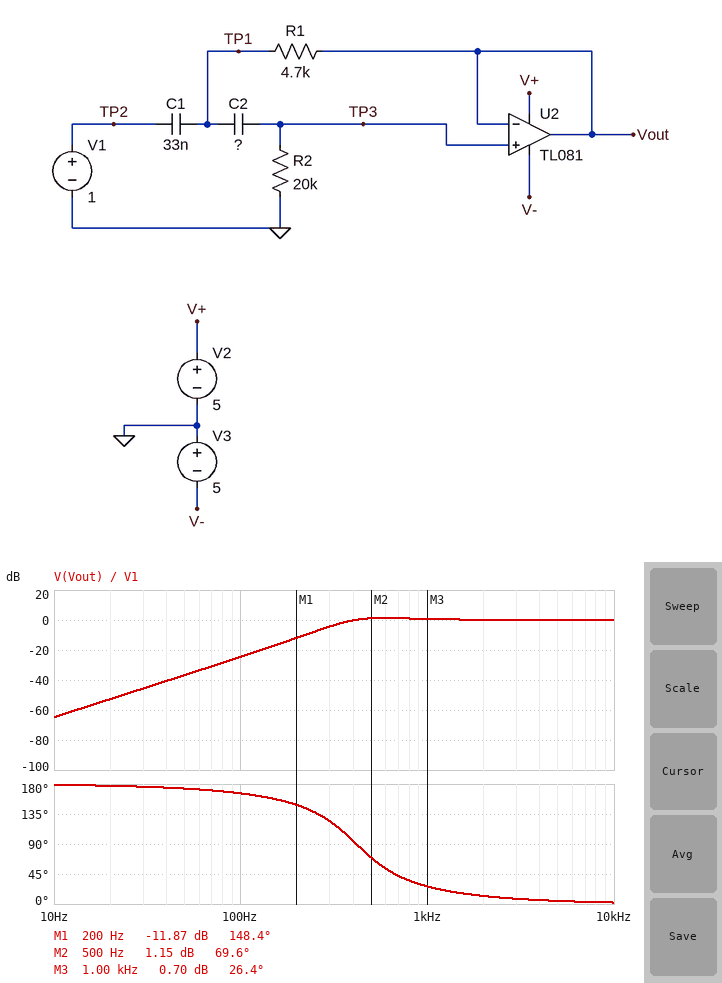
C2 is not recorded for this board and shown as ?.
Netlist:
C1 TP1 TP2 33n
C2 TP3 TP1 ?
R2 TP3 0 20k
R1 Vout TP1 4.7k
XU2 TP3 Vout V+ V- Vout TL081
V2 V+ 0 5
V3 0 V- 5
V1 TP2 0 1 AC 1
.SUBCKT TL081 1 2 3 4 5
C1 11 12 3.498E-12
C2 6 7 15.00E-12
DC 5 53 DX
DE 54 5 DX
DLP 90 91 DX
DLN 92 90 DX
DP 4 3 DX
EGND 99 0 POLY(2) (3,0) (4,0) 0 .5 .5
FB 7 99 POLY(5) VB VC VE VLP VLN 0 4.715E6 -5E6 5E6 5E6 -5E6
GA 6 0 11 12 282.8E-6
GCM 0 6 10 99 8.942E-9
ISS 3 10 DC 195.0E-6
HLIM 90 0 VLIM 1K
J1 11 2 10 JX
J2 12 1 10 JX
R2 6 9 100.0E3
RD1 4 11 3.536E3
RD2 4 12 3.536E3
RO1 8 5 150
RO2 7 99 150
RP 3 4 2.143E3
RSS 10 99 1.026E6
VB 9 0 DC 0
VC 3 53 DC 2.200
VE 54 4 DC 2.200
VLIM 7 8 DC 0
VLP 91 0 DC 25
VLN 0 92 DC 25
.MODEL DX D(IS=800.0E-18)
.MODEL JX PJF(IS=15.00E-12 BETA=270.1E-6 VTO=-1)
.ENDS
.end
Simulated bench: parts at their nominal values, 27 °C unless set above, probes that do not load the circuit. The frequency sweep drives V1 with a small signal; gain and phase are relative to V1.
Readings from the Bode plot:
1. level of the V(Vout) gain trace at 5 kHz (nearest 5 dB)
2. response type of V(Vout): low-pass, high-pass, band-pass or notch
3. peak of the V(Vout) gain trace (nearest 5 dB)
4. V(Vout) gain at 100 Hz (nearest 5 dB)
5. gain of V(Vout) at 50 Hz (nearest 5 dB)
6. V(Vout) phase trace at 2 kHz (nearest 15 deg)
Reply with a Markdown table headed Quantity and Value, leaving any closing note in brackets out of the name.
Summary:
| Quantity | Value |
|---|---|
| level of the V(Vout) gain trace at 5 kHz | 0 dB |
| response type of V(Vout): low-pass, high-pass, band-pass or notch | high-pass |
| peak of the V(Vout) gain trace | 0 dB |
| V(Vout) gain at 100 Hz | -25 dB |
| gain of V(Vout) at 50 Hz | -35 dB |
| V(Vout) phase trace at 2 kHz | 15 deg |
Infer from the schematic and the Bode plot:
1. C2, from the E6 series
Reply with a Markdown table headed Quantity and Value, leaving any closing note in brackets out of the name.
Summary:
| Quantity | Value |
|---|---|
| C2, from the E6 series | 47 nF |
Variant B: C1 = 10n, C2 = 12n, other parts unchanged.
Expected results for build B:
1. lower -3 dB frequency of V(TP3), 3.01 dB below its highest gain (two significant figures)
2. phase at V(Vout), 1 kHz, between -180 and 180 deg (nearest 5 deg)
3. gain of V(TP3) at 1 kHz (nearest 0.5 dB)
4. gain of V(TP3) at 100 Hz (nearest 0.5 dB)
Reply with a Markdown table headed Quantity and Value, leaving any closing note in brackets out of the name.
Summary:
| Quantity | Value |
|---|---|
| lower -3 dB frequency of V(TP3), 3.01 dB below its highest gain | 1.3 kHz |
| phase at V(Vout), 1 kHz, between -180 and 180 deg | 130 deg |
| gain of V(TP3) at 1 kHz | -5.5 dB |
| gain of V(TP3) at 100 Hz | -47.0 dB |
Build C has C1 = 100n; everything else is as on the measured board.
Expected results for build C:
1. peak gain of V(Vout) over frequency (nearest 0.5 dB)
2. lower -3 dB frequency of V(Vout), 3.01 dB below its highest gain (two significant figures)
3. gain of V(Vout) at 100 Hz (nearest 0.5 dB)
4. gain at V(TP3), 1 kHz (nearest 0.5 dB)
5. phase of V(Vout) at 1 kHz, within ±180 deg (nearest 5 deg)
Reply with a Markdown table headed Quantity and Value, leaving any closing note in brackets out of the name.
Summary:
| Quantity | Value |
|---|---|
| peak gain of V(Vout) over frequency | 1.0 dB |
| lower -3 dB frequency of V(Vout), 3.01 dB below its highest gain | 210 Hz |
| gain of V(Vout) at 100 Hz | -14.5 dB |
| gain at V(TP3), 1 kHz | 0 dB |
| phase of V(Vout) at 1 kHz, within ±180 deg | 15 deg |
